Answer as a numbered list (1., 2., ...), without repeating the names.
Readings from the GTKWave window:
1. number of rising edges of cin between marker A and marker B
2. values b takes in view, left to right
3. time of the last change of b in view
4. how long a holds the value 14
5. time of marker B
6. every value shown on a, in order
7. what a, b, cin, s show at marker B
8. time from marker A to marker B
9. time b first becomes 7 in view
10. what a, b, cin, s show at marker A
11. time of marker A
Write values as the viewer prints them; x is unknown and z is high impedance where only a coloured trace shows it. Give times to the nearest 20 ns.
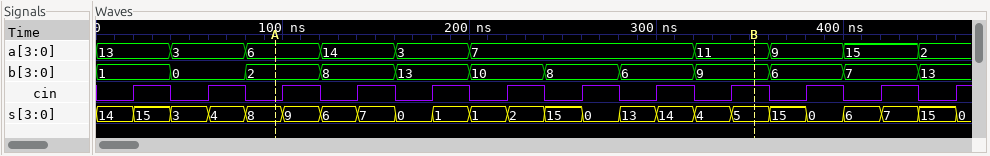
1. 7
2. 1, 0, 2, 8, 13, 10, 8, 6, 9, 6, 7, 13
3. 440 ns
4. 40 ns
5. 360 ns
6. 13, 3, 6, 14, 3, 7, 11, 9, 15, 2
7. a=11, b=9, cin=1, s=5
8. 260 ns
9. 400 ns
10. a=6, b=2, cin=0, s=8
11. 100 ns
